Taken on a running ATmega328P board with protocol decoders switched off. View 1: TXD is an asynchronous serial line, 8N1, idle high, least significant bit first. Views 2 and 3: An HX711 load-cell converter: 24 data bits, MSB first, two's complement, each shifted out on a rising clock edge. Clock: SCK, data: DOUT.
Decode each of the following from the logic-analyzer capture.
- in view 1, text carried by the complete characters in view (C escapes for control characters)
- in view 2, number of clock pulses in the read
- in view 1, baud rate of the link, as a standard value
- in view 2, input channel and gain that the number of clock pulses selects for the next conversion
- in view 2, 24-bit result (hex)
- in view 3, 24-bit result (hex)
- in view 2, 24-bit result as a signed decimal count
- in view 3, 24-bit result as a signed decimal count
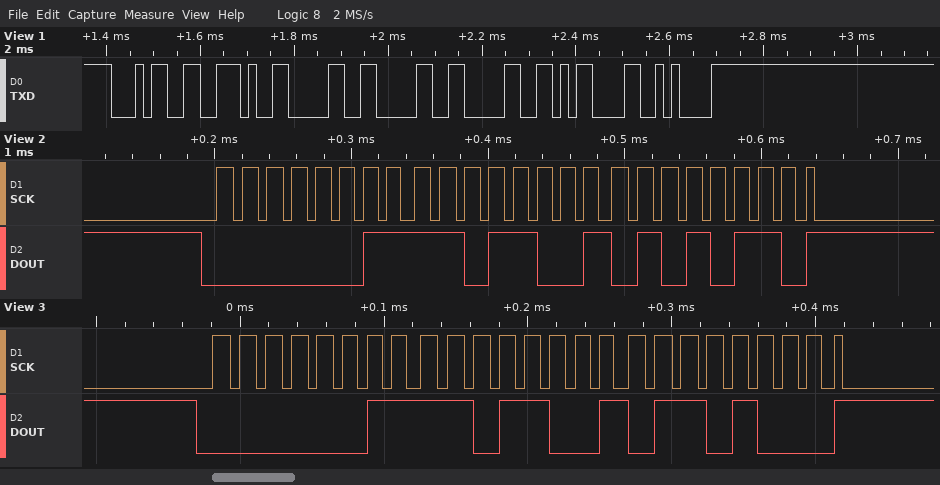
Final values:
"4.000\r\n"
25
57600 baud
channel A, gain 128
0x03D956
0x03D968
252246
252264
